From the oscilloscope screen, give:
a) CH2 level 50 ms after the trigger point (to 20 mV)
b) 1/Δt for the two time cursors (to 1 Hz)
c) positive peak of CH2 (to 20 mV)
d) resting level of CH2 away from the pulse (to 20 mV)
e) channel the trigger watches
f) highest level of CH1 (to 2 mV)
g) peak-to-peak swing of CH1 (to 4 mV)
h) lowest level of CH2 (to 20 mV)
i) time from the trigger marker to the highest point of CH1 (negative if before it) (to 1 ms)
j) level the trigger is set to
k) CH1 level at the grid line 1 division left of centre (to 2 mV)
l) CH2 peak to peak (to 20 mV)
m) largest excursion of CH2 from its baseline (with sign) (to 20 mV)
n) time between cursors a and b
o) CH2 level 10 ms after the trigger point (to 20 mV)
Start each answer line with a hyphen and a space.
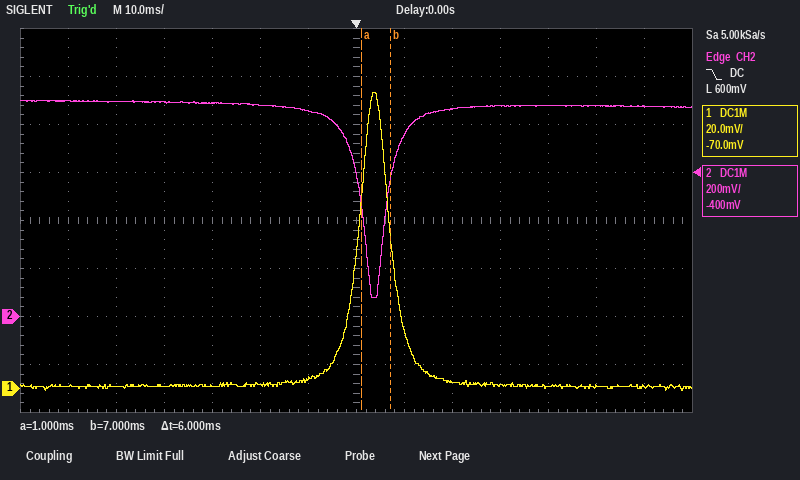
- 880 mV
- 167 Hz
- 900 mV
- 880 mV
- CH2
- 124 mV
- 124 mV
- 80 mV
- +4 ms
- 600 mV
- 4 mV
- 820 mV
- -800 mV
- 6 ms
- 760 mV
